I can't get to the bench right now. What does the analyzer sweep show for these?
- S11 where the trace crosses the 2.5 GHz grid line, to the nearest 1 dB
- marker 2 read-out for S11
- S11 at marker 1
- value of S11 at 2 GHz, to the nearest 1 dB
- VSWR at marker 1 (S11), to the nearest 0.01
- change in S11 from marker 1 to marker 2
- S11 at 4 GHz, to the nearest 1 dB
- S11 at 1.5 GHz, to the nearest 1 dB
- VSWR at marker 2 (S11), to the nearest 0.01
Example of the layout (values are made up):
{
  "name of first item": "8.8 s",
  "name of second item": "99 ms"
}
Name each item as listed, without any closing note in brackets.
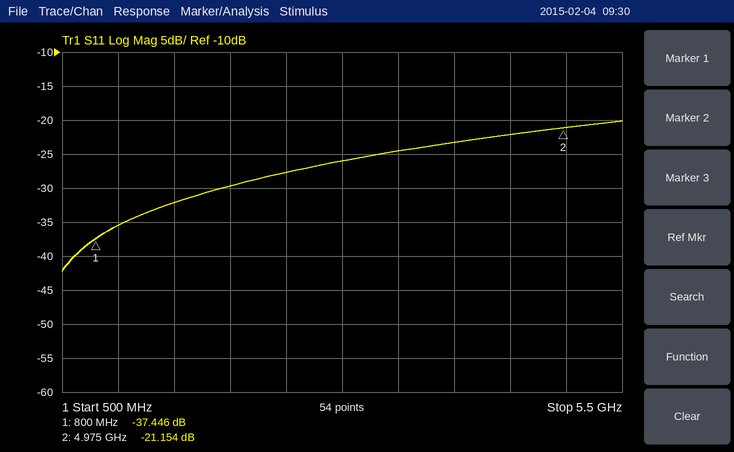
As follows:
{
  "S11 where the trace crosses the 2.5 GHz grid line, to the nearest 1 dB": "-28 dB",
  "marker 2 read-out for S11": "-21.154 dB",
  "S11 at marker 1": "-37.446 dB",
  "value of S11 at 2 GHz, to the nearest 1 dB": "-30 dB",
  "VSWR at marker 1 (S11), to the nearest 0.01": "1.03",
  "change in S11 from marker 1 to marker 2": "16.292 dB",
  "S11 at 4 GHz, to the nearest 1 dB": "-23 dB",
  "S11 at 1.5 GHz, to the nearest 1 dB": "-32 dB",
  "VSWR at marker 2 (S11), to the nearest 0.01": "1.19"
}
